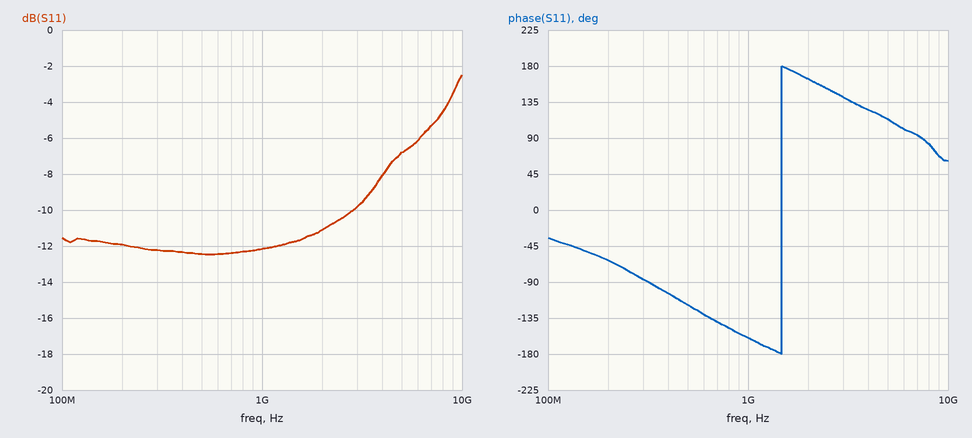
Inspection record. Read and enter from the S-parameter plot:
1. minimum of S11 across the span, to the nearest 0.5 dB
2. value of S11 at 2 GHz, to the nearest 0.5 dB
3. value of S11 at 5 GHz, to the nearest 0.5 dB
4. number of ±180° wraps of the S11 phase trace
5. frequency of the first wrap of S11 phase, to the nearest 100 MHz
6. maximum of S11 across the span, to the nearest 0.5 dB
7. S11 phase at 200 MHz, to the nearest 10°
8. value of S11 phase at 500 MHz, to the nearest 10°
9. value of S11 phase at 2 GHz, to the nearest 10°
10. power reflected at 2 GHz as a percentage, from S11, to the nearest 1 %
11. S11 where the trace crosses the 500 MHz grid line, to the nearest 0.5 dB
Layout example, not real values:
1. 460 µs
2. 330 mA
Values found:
1. -12.5 dB
2. -11.0 dB
3. -7.0 dB
4. 1
5. 1.5 GHz
6. -2.5 dB
7. -60°
8. -120°
9. 160°
10. 8 %
11. -12.5 dB
